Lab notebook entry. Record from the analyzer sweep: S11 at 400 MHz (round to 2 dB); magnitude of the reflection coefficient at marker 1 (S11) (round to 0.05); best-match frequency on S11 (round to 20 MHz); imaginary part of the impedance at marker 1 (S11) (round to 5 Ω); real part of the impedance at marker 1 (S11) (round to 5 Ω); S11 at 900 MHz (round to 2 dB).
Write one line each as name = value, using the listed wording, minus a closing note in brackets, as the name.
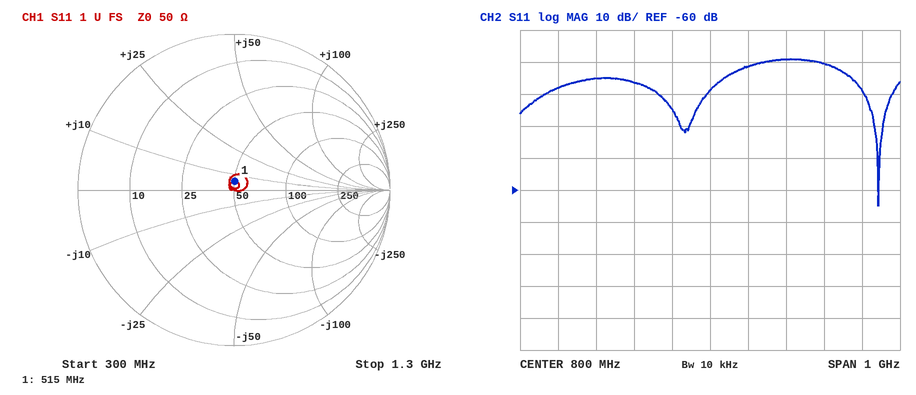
S11 at 400 MHz = -28 dB
magnitude of the reflection coefficient at marker 1 (S11) = 0.05
best-match frequency on S11 = 1.24 GHz
imaginary part of the impedance at marker 1 (S11) = +5 Ω
real part of the impedance at marker 1 (S11) = 50 Ω
S11 at 900 MHz = -22 dB
